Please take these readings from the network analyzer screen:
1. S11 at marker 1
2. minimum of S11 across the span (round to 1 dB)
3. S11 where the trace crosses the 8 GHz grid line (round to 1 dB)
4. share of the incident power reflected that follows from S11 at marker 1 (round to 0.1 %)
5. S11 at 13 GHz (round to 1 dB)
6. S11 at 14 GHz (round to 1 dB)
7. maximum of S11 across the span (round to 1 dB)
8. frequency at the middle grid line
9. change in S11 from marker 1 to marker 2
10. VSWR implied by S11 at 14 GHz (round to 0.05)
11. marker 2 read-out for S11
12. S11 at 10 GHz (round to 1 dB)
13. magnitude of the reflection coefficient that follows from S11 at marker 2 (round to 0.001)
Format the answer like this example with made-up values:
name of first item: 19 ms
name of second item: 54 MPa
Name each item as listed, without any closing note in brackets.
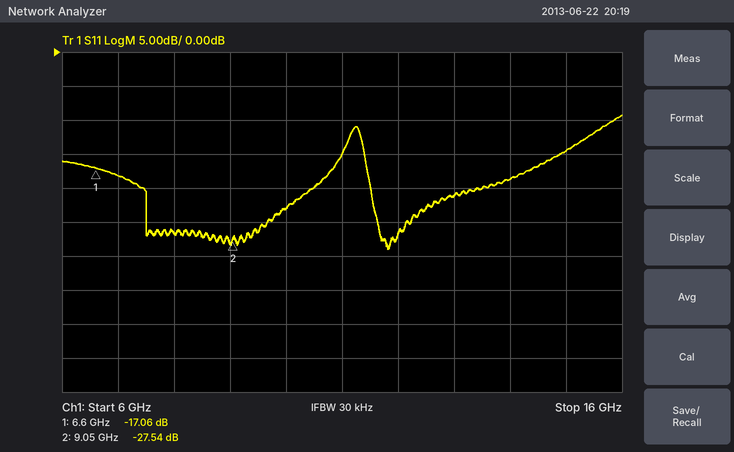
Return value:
S11 at marker 1: -17.06 dB
minimum of S11 across the span: -29 dB
S11 where the trace crosses the 8 GHz grid line: -27 dB
share of the incident power reflected that follows from S11 at marker 1: 2.0 %
S11 at 13 GHz: -21 dB
S11 at 14 GHz: -19 dB
maximum of S11 across the span: -9 dB
frequency at the middle grid line: 11 GHz
change in S11 from marker 1 to marker 2: -10.48 dB
VSWR implied by S11 at 14 GHz: 1.25
marker 2 read-out for S11: -27.54 dB
S11 at 10 GHz: -23 dB
magnitude of the reflection coefficient that follows from S11 at marker 2: 0.042
